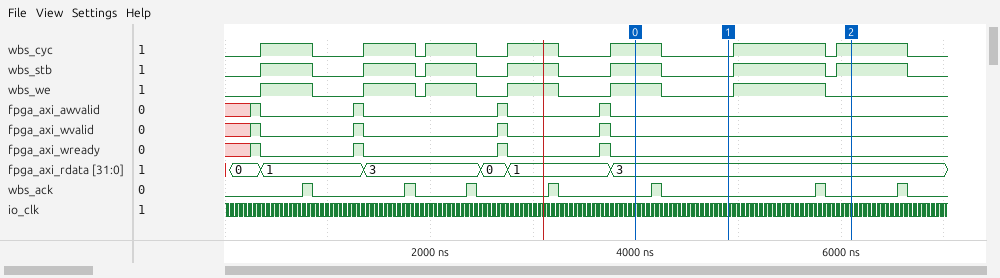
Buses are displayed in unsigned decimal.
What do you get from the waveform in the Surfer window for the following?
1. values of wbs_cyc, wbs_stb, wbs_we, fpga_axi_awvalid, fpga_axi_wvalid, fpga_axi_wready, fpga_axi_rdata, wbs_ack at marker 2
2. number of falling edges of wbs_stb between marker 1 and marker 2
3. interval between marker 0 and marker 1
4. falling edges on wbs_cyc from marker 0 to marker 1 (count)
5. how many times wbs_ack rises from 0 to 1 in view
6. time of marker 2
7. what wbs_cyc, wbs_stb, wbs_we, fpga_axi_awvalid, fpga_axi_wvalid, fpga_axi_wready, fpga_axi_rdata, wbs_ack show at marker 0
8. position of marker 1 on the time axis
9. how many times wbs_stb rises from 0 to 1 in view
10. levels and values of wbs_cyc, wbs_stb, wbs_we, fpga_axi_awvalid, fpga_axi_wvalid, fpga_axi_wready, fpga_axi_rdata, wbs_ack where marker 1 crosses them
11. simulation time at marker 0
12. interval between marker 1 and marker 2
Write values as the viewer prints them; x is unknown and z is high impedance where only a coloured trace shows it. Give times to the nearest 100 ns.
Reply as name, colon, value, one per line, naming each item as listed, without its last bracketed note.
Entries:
values of wbs_cyc, wbs_stb, wbs_we, fpga_axi_awvalid, fpga_axi_wvalid, fpga_axi_wready, fpga_axi_rdata, wbs_ack at marker 2: wbs_cyc=1, wbs_stb=1, wbs_we=0, fpga_axi_awvalid=0, fpga_axi_wvalid=0, fpga_axi_wready=0, fpga_axi_rdata=3, wbs_ack=0
number of falling edges of wbs_stb between marker 1 and marker 2: 1
interval between marker 0 and marker 1: 900 ns
falling edges on wbs_cyc from marker 0 to marker 1: 1
how many times wbs_ack rises from 0 to 1 in view: 7
time of marker 2: 6100 ns
what wbs_cyc, wbs_stb, wbs_we, fpga_axi_awvalid, fpga_axi_wvalid, fpga_axi_wready, fpga_axi_rdata, wbs_ack show at marker 0: wbs_cyc=1, wbs_stb=1, wbs_we=1, fpga_axi_awvalid=0, fpga_axi_wvalid=0, fpga_axi_wready=0, fpga_axi_rdata=3, wbs_ack=0
position of marker 1 on the time axis: 4900 ns
how many times wbs_stb rises from 0 to 1 in view: 7
levels and values of wbs_cyc, wbs_stb, wbs_we, fpga_axi_awvalid, fpga_axi_wvalid, fpga_axi_wready, fpga_axi_rdata, wbs_ack where marker 1 crosses them: wbs_cyc=0, wbs_stb=0, wbs_we=0, fpga_axi_awvalid=0, fpga_axi_wvalid=0, fpga_axi_wready=0, fpga_axi_rdata=3, wbs_ack=0
simulation time at marker 0: 4000 ns
interval between marker 1 and marker 2: 1200 ns
